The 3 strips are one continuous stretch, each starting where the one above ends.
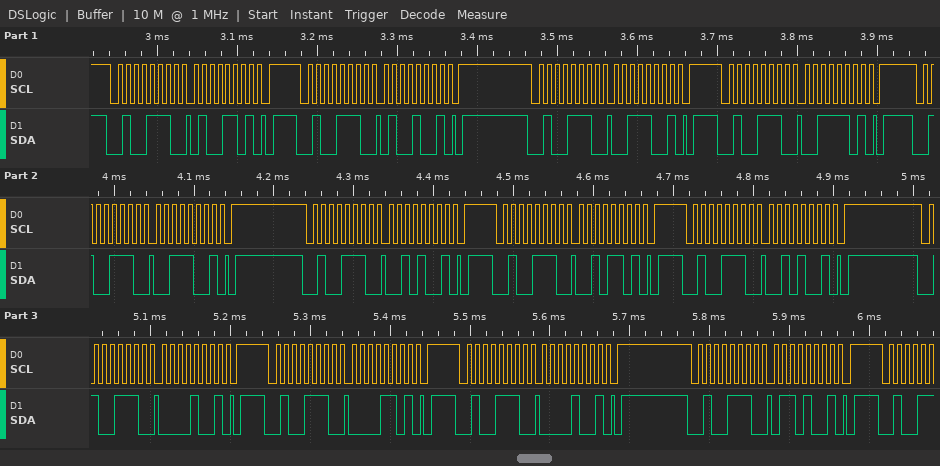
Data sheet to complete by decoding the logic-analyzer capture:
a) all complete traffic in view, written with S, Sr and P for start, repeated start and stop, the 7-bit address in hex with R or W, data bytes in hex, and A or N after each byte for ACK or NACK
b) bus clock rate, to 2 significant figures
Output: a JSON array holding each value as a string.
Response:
["S 27W A 4D A P S 27W A 49 A P S 27W A 39 A P S 27W A 3D A P S 27W A 39 A P S 27W A 29 A P S 27W A 2D A P S 27W A 29 A P S 27W A 09 A P S 27W A 0D A P S 27W A 09 A P S 27W A 69 A P", "100 kHz"]
